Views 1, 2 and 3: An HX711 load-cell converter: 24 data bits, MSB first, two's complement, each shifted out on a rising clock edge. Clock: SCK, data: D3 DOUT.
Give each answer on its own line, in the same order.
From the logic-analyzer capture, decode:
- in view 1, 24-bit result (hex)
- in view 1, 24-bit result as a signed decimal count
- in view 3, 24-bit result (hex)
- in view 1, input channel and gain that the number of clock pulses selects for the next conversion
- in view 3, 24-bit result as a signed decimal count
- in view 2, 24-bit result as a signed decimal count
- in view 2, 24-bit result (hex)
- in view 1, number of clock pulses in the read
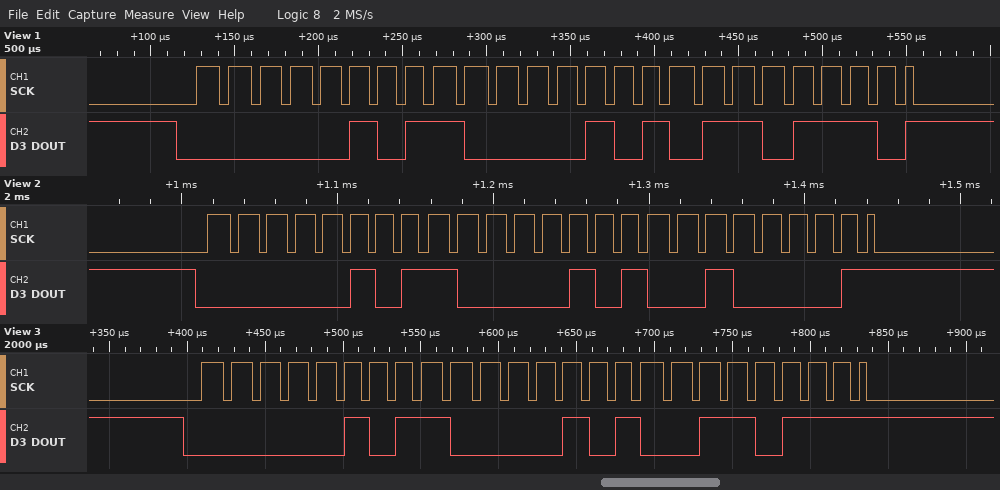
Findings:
0x05856E
361838
0x058537
channel A, gain 128
361783
361761
0x058521
25
